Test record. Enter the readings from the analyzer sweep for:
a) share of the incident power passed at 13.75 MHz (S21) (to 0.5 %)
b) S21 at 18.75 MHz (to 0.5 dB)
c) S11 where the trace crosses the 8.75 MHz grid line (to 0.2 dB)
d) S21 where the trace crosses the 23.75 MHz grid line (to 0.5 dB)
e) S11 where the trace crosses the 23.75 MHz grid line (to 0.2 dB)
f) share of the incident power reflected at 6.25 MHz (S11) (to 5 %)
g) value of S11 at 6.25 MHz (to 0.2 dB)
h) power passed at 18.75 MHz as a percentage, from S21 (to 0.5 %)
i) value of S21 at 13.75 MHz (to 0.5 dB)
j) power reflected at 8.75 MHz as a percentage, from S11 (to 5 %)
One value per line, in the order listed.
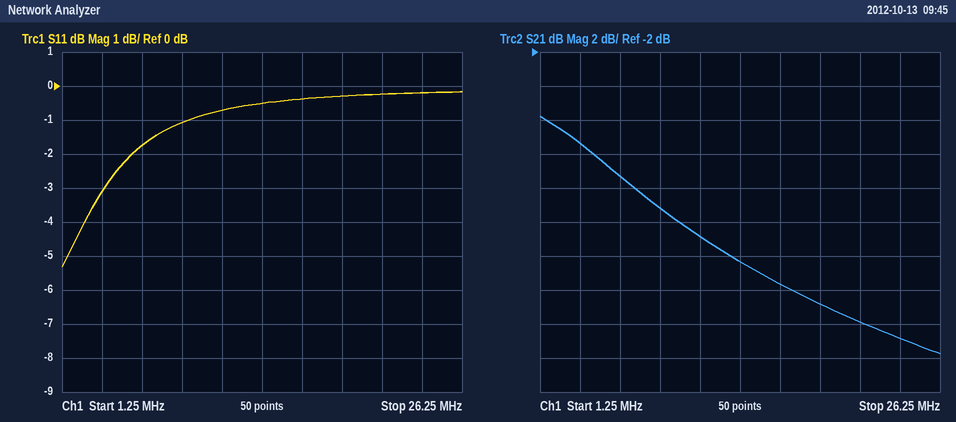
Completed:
3.5 %
-17.0 dB
-1.0 dB
-19.0 dB
-0.2 dB
65 %
-1.8 dB
2.0 %
-14.5 dB
80 %
